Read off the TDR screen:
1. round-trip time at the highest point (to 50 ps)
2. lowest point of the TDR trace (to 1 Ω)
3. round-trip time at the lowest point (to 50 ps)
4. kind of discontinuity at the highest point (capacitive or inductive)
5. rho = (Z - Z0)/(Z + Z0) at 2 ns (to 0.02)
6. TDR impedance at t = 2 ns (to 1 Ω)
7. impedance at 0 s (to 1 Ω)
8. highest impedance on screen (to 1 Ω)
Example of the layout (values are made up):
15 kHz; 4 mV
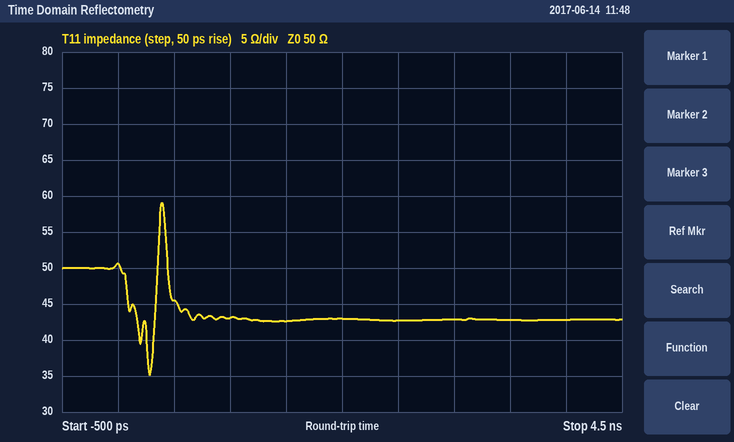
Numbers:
400 ps; 35 Ω; 300 ps; inductive; -0.08; 43 Ω; 51 Ω; 59 Ω
